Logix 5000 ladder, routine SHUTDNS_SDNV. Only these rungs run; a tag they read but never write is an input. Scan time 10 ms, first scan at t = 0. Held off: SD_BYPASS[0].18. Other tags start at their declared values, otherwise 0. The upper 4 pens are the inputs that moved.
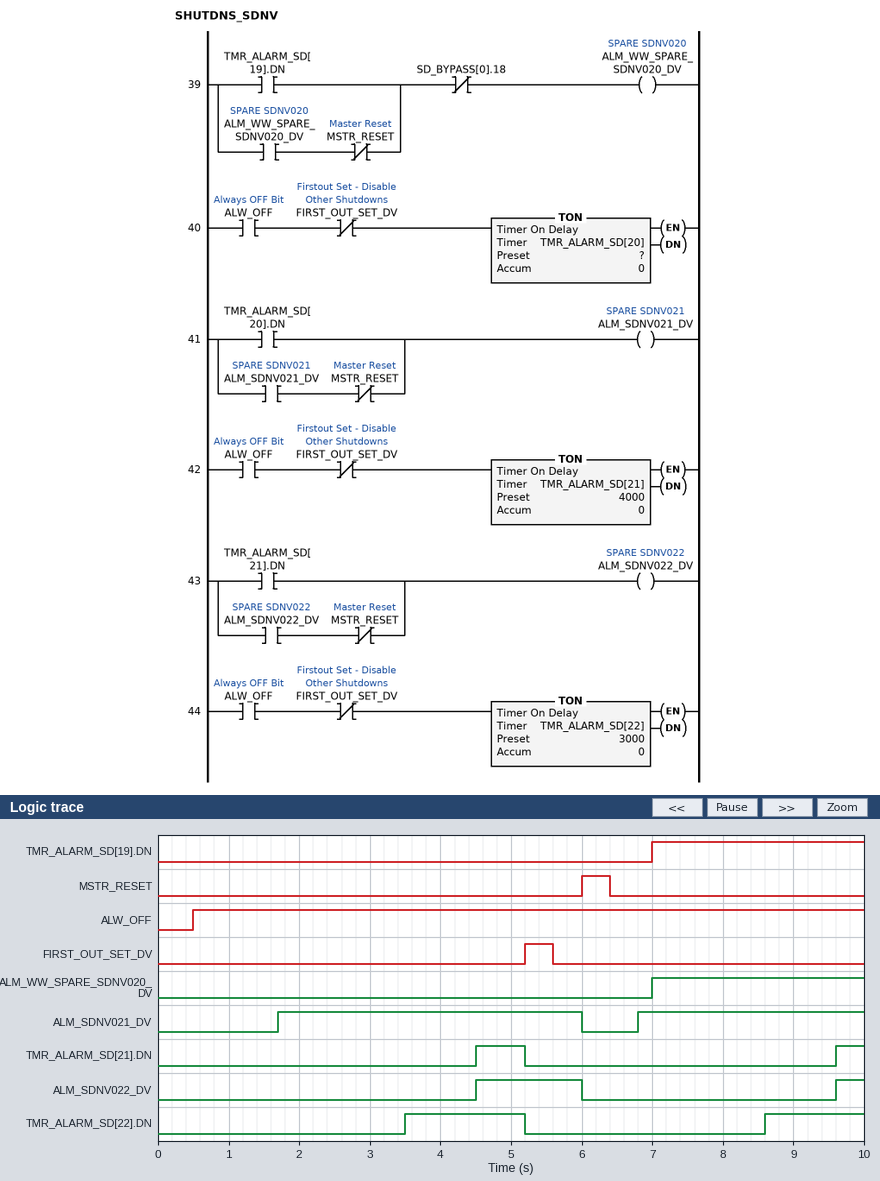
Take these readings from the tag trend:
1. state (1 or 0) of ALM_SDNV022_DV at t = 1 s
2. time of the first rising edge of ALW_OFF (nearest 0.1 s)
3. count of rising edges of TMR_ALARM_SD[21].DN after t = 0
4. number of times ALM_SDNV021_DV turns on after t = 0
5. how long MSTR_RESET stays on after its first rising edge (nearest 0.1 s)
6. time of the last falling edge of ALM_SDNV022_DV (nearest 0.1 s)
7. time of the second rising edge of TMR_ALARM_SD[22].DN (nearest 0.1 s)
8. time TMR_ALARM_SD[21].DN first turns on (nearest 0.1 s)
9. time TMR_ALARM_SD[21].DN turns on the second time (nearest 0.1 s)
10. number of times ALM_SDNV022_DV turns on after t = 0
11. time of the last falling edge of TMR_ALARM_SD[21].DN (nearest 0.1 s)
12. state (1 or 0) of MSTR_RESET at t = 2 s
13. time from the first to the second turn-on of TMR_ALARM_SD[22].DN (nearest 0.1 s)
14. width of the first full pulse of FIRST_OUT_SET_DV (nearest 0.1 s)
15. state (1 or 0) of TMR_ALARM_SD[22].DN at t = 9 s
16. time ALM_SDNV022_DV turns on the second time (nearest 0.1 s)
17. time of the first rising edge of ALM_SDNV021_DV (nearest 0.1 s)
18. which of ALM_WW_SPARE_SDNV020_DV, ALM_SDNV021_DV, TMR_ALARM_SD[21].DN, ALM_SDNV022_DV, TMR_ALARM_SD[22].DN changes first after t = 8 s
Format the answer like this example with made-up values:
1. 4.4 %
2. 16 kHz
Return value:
1. 0
2. 0.5 s
3. 2
4. 2
5. 0.4 s
6. 6.0 s
7. 8.6 s
8. 4.5 s
9. 9.6 s
10. 2
11. 5.2 s
12. 0
13. 5.1 s
14. 0.4 s
15. 1
16. 9.6 s
17. 1.7 s
18. TMR_ALARM_SD[22].DN
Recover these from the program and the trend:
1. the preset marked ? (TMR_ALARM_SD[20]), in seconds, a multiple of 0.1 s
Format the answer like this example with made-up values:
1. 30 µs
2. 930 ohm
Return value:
1. 1.2 s
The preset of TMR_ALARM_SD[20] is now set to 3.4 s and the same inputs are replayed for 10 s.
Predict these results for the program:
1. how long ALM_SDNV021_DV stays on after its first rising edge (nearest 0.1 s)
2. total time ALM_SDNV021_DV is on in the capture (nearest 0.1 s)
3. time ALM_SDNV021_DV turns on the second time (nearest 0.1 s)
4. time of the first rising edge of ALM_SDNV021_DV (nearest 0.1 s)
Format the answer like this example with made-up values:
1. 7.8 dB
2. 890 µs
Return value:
1. 2.1 s
2. 3.1 s
3. 9.0 s
4. 3.9 s
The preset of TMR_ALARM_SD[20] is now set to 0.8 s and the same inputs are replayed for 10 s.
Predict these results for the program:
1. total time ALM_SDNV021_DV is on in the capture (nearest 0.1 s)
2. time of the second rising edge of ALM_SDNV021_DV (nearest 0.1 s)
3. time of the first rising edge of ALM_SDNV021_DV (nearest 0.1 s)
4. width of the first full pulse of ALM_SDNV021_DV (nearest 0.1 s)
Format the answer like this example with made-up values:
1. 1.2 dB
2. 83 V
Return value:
1. 8.3 s
2. 6.4 s
3. 1.3 s
4. 4.7 s
